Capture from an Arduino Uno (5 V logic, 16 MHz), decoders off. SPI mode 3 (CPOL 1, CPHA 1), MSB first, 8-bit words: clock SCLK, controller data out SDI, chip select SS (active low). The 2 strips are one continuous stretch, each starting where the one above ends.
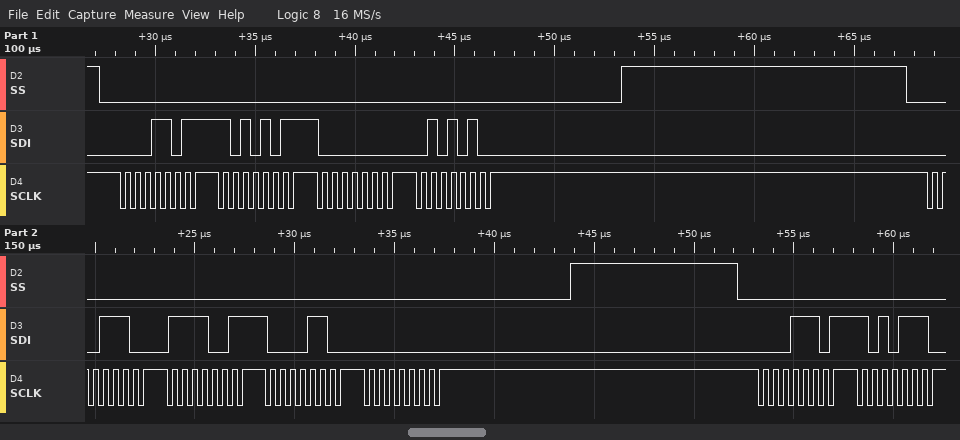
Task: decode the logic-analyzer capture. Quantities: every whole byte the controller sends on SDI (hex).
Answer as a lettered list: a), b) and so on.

a) 1B AB 00 54 1C F3 0C 00 1D AE
